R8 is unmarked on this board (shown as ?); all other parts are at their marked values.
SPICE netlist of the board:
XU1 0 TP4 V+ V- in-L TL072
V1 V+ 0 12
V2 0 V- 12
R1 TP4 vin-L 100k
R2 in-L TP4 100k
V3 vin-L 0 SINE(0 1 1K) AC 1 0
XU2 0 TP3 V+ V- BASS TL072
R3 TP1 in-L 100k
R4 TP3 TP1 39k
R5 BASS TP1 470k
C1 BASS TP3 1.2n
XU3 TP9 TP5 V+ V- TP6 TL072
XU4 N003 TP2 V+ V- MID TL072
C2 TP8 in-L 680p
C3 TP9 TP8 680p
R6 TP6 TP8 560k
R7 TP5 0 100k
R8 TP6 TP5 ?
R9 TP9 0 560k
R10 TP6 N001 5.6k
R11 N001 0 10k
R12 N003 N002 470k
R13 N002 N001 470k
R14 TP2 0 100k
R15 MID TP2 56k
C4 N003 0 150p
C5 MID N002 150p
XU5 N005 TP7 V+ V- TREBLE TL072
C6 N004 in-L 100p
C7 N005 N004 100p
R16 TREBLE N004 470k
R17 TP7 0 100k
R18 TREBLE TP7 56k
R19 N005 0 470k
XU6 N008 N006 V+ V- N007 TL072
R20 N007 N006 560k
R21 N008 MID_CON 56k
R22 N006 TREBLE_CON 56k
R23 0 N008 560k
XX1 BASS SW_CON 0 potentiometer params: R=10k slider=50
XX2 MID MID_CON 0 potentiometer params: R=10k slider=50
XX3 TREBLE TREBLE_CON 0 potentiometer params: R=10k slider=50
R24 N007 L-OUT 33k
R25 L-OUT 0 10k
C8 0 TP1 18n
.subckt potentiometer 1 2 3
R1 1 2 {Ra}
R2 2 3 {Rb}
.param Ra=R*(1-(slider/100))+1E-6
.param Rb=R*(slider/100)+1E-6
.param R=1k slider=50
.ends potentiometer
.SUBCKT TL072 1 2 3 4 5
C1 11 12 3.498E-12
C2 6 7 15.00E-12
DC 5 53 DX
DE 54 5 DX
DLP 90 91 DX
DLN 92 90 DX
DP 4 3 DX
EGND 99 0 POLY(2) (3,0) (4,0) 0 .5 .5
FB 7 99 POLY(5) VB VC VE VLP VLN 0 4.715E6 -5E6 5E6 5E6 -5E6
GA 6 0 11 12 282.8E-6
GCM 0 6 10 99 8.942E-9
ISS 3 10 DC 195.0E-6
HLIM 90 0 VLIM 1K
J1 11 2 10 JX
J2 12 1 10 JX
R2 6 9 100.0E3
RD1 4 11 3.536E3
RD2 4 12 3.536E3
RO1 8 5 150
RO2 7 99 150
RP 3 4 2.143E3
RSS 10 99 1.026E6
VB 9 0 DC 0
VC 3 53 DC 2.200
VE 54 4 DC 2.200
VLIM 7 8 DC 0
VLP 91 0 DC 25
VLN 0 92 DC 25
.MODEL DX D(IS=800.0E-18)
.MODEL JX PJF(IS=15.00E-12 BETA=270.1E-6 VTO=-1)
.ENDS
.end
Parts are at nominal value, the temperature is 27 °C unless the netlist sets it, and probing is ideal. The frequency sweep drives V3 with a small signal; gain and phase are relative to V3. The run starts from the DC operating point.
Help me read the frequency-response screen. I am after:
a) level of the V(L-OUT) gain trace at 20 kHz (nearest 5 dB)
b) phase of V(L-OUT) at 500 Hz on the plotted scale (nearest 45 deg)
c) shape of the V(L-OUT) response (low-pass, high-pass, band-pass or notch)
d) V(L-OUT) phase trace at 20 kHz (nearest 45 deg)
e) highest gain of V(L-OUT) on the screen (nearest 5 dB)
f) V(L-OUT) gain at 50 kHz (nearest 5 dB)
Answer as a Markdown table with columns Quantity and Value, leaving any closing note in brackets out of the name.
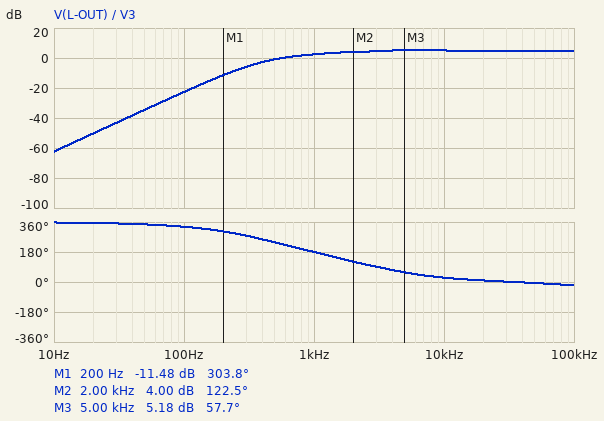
| Quantity | Value |
|---|---|
| level of the V(L-OUT) gain trace at 20 kHz | 5 dB |
| phase of V(L-OUT) at 500 Hz on the plotted scale | 225 deg |
| shape of the V(L-OUT) response | high-pass |
| V(L-OUT) phase trace at 20 kHz | 0 deg |
| highest gain of V(L-OUT) on the screen | 5 dB |
| V(L-OUT) gain at 50 kHz | 5 dB |
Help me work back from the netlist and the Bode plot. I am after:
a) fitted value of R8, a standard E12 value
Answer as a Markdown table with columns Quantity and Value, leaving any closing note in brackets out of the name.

| Quantity | Value |
|---|---|
| fitted value of R8, a standard E12 value | 22 kΩ |
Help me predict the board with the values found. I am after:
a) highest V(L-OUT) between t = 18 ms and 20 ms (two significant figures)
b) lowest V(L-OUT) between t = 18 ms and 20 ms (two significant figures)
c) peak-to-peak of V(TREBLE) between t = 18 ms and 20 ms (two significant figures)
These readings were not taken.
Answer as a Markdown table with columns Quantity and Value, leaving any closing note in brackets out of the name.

| Quantity | Value |
|---|---|
| highest V(L-OUT) between t = 18 ms and 20 ms | 1.3 V |
| lowest V(L-OUT) between t = 18 ms and 20 ms | -1.3 V |
| peak-to-peak of V(TREBLE) between t = 18 ms and 20 ms | 270 mV |
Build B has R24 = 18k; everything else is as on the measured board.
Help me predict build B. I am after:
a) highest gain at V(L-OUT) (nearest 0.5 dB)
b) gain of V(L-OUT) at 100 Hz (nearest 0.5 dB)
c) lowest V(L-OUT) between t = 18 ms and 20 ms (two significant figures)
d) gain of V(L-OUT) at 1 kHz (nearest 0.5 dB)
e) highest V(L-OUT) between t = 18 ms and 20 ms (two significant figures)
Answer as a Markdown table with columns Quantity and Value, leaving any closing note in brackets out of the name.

| Quantity | Value |
|---|---|
| highest gain at V(L-OUT) | 9.0 dB |
| gain of V(L-OUT) at 100 Hz | -19.0 dB |
| lowest V(L-OUT) between t = 18 ms and 20 ms | -2.0 V |
| gain of V(L-OUT) at 1 kHz | 6.0 dB |
| highest V(L-OUT) between t = 18 ms and 20 ms | 2.0 V |
